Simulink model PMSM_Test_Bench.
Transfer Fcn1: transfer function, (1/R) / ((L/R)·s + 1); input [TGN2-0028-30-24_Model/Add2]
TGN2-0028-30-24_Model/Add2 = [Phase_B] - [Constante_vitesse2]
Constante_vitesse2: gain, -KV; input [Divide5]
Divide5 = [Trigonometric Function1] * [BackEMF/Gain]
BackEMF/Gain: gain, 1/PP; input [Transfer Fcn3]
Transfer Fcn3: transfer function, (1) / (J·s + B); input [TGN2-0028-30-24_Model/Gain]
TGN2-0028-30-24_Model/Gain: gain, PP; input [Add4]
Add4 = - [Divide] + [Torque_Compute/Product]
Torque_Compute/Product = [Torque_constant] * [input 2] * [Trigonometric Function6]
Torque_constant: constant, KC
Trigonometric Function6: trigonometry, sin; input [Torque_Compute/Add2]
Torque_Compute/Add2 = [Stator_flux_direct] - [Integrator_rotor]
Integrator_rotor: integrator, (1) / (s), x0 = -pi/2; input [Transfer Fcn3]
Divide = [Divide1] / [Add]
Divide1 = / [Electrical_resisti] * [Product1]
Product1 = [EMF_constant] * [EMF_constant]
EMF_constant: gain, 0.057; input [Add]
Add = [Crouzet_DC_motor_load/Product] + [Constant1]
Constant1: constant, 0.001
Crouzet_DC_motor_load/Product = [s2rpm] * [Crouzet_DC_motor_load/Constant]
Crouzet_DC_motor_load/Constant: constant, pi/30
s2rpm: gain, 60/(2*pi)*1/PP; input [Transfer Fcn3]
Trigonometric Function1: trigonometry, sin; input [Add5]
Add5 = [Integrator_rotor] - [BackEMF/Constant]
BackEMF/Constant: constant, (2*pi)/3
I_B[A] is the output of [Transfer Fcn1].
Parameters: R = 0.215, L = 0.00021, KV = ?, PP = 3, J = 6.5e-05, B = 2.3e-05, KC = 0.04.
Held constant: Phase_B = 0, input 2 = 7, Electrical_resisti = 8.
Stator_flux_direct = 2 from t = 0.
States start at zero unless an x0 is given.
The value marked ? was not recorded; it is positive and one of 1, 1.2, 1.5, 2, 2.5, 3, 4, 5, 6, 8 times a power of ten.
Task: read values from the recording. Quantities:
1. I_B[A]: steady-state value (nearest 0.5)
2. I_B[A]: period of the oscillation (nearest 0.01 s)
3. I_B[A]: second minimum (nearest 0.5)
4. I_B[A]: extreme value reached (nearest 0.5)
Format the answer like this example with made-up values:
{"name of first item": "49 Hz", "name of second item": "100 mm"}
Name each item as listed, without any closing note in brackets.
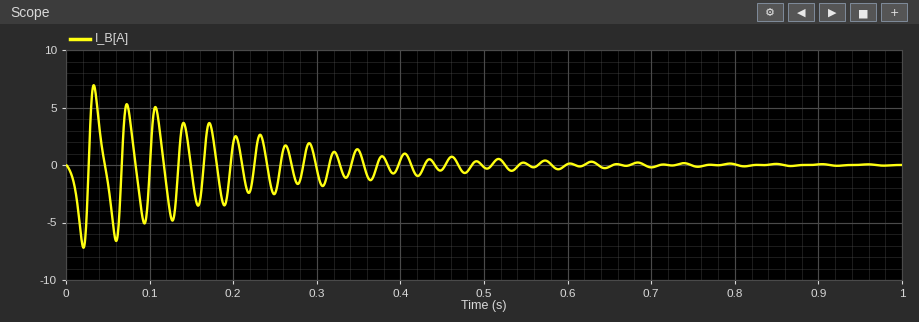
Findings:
{"I_B[A]: steady-state value": "0.0", "I_B[A]: period of the oscillation": "0.04 s", "I_B[A]: second minimum": "-6.5", "I_B[A]: extreme value reached": "-7.0"}
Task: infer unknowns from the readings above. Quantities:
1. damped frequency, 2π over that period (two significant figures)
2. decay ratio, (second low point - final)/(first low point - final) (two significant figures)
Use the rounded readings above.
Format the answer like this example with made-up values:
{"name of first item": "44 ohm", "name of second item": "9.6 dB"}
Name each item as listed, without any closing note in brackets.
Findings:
{"damped frequency, 2π over that period": "160 rad/s", "decay ratio, (second low point - final)/(first low point - final)": "0.93"}
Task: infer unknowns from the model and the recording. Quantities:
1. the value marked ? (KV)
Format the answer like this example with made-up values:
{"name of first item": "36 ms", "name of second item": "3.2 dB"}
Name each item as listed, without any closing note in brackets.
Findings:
{"the value marked ?": "0.03"}
